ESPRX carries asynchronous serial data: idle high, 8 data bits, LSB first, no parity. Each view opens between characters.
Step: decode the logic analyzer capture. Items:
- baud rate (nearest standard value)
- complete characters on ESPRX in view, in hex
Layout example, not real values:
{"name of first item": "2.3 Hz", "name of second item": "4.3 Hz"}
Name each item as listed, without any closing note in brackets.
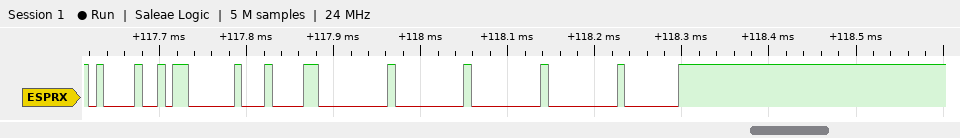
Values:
{"baud rate": "115200 baud", "complete characters on ESPRX in view, in hex": "21, 03, 84, 00, 00, 00, 00, C0"}
